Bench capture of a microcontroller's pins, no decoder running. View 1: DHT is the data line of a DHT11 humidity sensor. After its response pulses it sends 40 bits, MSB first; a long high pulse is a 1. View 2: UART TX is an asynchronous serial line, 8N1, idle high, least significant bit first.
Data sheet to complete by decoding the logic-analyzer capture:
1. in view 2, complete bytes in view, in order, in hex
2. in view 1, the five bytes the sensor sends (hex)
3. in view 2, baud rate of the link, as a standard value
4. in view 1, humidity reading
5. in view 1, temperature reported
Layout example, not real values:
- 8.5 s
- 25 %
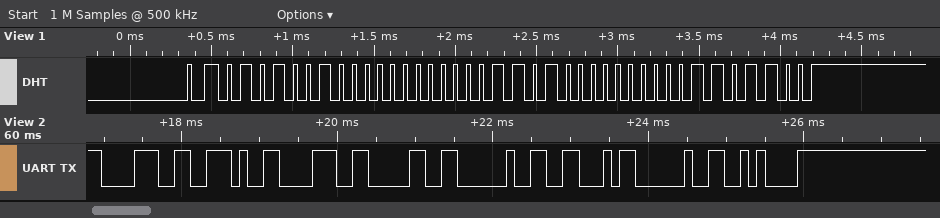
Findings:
- 38 2E 38 30 20 46 20 0A
- 52 00 1A 00 6C
- 9600 baud
- 82 %
- 26.0 °C
